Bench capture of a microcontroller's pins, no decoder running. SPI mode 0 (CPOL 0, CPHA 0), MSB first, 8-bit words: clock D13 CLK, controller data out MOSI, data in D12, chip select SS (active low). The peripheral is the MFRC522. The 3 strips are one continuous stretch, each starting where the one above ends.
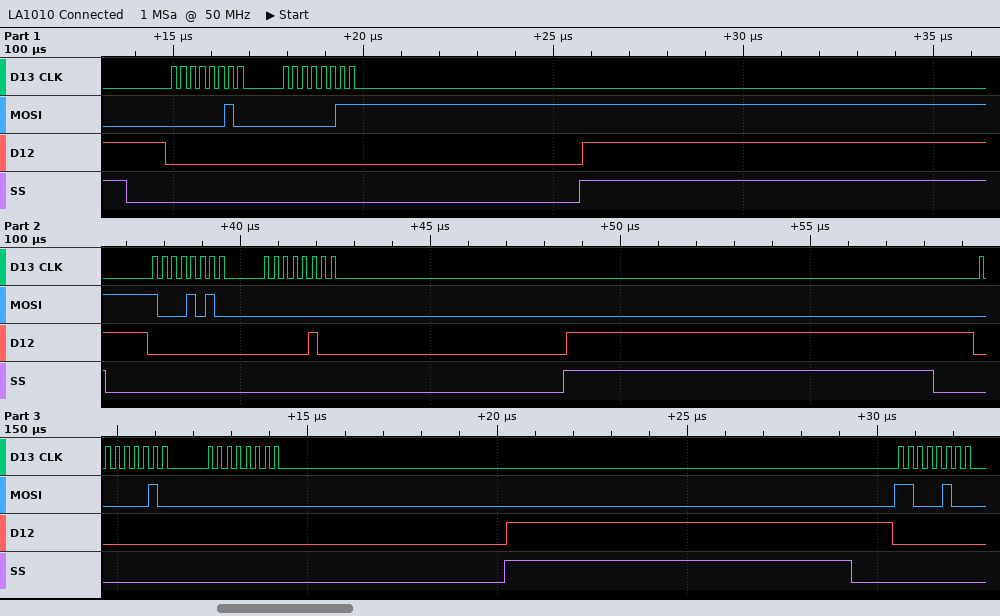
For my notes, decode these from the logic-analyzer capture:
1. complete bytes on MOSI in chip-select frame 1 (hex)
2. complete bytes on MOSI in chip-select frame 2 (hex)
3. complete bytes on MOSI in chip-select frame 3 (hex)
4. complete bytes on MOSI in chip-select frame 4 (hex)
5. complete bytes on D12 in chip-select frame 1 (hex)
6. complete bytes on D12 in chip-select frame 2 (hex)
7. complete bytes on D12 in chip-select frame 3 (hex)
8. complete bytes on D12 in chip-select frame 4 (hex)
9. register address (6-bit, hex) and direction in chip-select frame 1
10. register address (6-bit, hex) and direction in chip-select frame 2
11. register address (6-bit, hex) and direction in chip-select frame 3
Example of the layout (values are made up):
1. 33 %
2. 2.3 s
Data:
1. 0x02 0x03
2. 0x8A 0x00
3. 0x02 0x00
4. 0xC4
5. 0x00 0x00
6. 0x00 0x04
7. 0x00 0x00
8. 0x00
9. 0x01 write
10. 0x05 read
11. 0x01 write
